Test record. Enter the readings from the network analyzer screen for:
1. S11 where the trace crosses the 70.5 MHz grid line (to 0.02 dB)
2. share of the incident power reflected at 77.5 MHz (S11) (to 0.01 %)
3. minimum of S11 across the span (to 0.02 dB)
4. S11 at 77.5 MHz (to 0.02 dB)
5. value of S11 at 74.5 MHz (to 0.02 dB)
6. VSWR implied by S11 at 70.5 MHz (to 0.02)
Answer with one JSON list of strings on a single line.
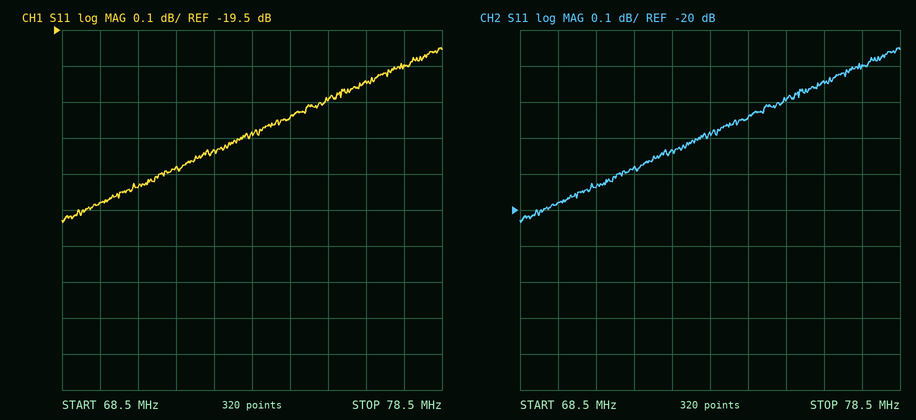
["-19.94 dB", "1.10 %", "-20.04 dB", "-19.60 dB", "-19.74 dB", "1.22"]
